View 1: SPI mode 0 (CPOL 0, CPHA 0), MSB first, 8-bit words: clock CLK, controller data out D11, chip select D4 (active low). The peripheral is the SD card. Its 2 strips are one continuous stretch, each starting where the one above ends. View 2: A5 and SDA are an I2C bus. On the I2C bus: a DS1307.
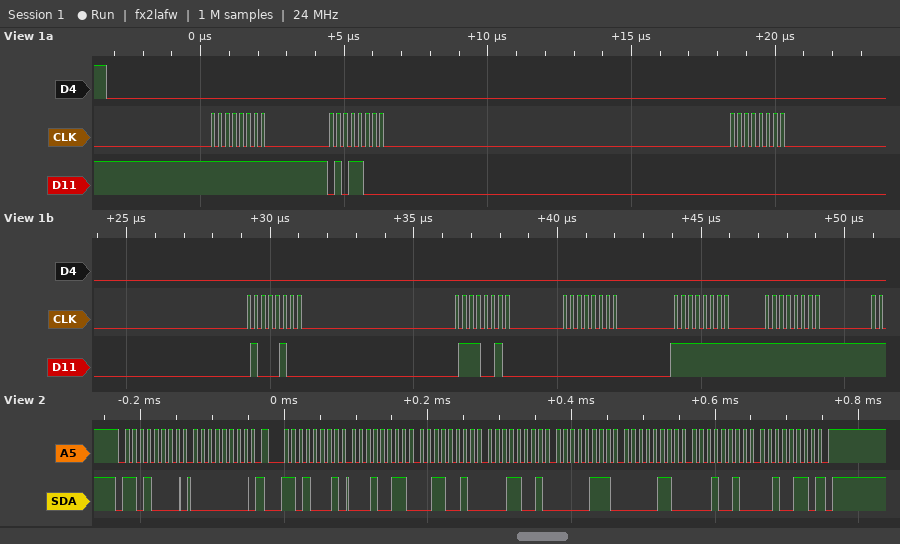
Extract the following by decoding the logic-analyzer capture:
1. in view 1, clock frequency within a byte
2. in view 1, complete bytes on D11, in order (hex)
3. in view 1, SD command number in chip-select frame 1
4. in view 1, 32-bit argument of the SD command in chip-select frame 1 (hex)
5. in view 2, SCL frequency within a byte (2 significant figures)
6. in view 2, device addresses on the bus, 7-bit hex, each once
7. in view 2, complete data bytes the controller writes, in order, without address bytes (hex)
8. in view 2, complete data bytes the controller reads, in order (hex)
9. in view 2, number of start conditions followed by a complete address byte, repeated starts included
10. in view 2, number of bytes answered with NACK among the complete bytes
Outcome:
4 MHz
FF 58 00 44 72 00 FF FF
CMD24
0x00447200
100 kHz
0x68
00
13 32 19 07 06 12 26
2
1
